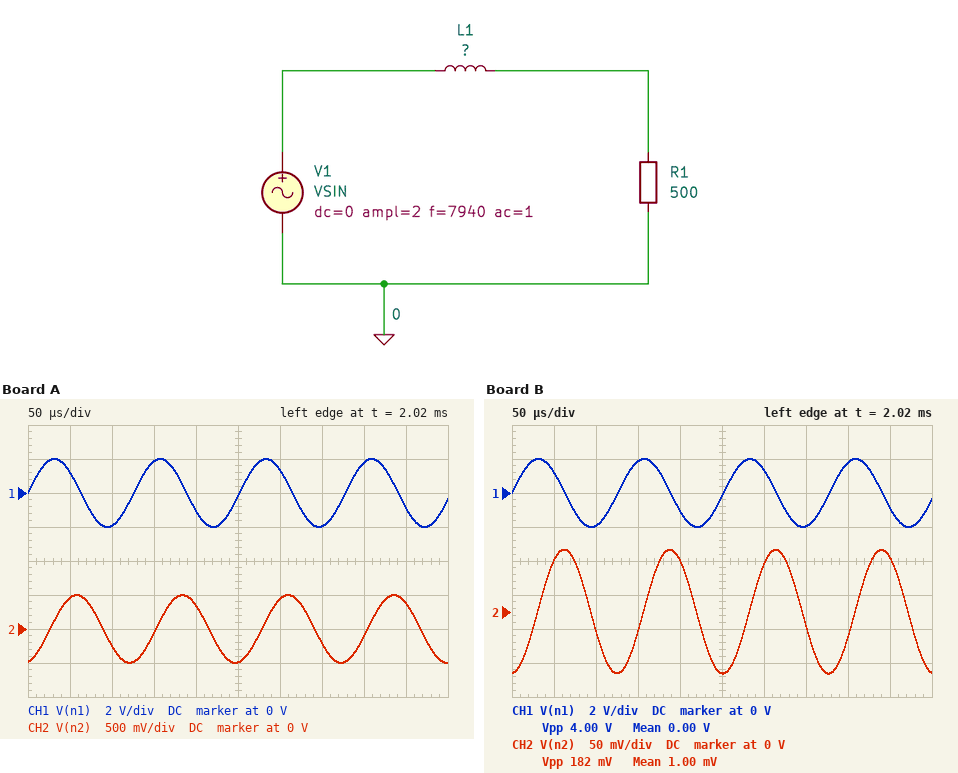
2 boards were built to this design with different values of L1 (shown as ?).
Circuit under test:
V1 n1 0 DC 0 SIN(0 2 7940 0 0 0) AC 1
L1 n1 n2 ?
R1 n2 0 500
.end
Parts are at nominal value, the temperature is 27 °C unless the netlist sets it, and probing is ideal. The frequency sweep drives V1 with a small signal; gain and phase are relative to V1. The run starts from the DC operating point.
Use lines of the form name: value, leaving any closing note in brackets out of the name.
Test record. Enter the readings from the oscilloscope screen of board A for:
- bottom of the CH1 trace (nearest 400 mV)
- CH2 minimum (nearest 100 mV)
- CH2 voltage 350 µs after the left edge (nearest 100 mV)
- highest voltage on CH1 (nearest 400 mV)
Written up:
bottom of the CH1 trace: -2.0 V
CH2 minimum: -500 mV
CH2 voltage 350 µs after the left edge: -200 mV
highest voltage on CH1: 2.0 V
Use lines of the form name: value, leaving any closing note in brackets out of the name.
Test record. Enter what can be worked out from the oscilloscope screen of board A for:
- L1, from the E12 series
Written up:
L1, from the E12 series: 39 mH
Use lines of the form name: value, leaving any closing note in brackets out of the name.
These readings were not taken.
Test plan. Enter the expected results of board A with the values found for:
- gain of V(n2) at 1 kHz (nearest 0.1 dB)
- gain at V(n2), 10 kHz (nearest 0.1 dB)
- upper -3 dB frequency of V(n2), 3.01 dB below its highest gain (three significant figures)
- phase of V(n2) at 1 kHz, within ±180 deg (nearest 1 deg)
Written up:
gain of V(n2) at 1 kHz: -0.9 dB
gain at V(n2), 10 kHz: -14.0 dB
upper -3 dB frequency of V(n2), 3.01 dB below its highest gain: 2.04 kHz
phase of V(n2) at 1 kHz, within ±180 deg: -26 deg
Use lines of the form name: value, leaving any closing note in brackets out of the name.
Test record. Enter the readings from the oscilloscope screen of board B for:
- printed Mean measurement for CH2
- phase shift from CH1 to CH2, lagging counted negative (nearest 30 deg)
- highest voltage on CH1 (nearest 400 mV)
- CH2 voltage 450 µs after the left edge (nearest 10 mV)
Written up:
printed Mean measurement for CH2: 1.00 mV
phase shift from CH1 to CH2, lagging counted negative: -90 deg
highest voltage on CH1: 2.0 V
CH2 voltage 450 µs after the left edge: 80 mV
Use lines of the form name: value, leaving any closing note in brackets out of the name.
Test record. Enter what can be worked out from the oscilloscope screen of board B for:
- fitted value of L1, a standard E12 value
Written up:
fitted value of L1, a standard E12 value: 220 mH
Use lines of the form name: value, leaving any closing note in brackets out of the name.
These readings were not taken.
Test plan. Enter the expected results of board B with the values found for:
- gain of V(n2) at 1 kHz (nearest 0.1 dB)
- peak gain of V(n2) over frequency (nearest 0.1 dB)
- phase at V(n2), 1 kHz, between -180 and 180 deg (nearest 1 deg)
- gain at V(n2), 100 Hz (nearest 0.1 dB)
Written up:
gain of V(n2) at 1 kHz: -9.4 dB
peak gain of V(n2) over frequency: 0 dB
phase at V(n2), 1 kHz, between -180 and 180 deg: -70 deg
gain at V(n2), 100 Hz: -0.3 dB
